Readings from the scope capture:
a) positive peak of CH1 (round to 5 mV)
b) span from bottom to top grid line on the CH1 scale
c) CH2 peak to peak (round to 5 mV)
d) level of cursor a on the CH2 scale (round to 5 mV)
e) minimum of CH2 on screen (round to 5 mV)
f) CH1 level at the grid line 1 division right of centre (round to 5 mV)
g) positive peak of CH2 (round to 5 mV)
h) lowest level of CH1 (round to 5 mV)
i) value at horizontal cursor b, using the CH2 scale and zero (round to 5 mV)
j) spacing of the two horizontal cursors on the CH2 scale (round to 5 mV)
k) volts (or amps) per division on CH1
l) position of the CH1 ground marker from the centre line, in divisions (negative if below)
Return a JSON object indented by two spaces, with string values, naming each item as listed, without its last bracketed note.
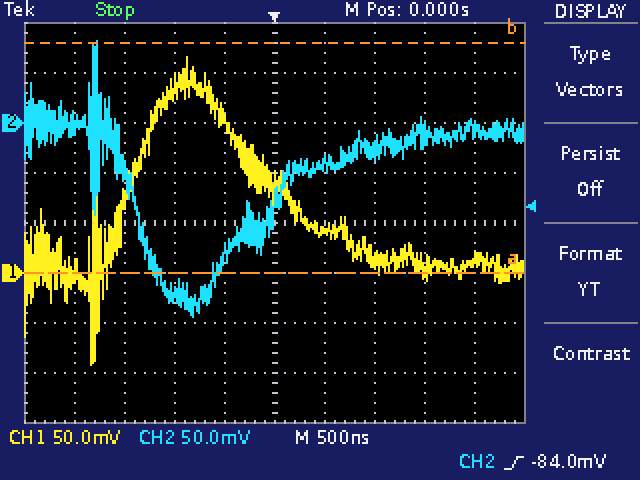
{
  "positive peak of CH1": "215 mV",
  "span from bottom to top grid line on the CH1 scale": "400 mV",
  "CH2 peak to peak": "275 mV",
  "level of cursor a on the CH2 scale": "-150 mV",
  "minimum of CH2 on screen": "-195 mV",
  "CH1 level at the grid line 1 division right of centre": "40 mV",
  "positive peak of CH2": "80 mV",
  "lowest level of CH1": "-90 mV",
  "value at horizontal cursor b, using the CH2 scale and zero": "80 mV",
  "spacing of the two horizontal cursors on the CH2 scale": "230 mV",
  "volts (or amps) per division on CH1": "50 mV",
  "position of the CH1 ground marker from the centre line, in divisions": "-1.0 div"
}
